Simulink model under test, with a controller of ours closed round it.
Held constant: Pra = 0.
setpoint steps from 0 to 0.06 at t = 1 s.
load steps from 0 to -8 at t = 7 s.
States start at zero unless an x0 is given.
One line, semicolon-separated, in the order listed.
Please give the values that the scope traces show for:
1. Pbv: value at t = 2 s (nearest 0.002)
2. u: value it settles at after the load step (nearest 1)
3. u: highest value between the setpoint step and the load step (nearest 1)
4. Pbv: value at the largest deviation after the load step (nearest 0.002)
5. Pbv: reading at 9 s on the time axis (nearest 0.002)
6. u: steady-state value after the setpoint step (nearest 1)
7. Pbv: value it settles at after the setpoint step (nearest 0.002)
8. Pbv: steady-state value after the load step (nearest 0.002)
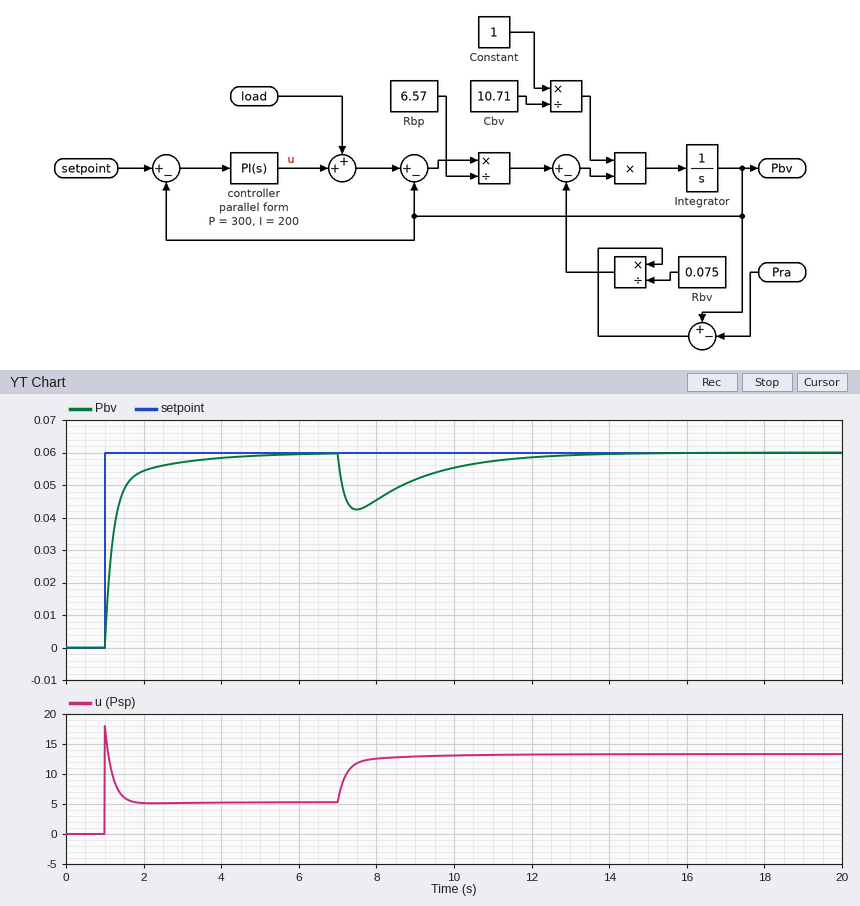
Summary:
0.054; 13; 18; 0.042; 0.052; 5; 0.060; 0.060
